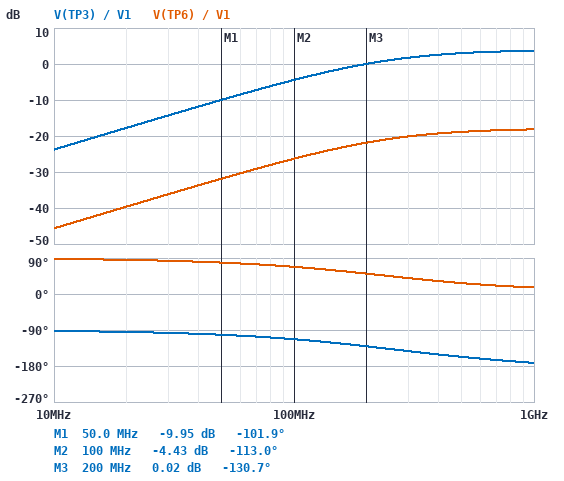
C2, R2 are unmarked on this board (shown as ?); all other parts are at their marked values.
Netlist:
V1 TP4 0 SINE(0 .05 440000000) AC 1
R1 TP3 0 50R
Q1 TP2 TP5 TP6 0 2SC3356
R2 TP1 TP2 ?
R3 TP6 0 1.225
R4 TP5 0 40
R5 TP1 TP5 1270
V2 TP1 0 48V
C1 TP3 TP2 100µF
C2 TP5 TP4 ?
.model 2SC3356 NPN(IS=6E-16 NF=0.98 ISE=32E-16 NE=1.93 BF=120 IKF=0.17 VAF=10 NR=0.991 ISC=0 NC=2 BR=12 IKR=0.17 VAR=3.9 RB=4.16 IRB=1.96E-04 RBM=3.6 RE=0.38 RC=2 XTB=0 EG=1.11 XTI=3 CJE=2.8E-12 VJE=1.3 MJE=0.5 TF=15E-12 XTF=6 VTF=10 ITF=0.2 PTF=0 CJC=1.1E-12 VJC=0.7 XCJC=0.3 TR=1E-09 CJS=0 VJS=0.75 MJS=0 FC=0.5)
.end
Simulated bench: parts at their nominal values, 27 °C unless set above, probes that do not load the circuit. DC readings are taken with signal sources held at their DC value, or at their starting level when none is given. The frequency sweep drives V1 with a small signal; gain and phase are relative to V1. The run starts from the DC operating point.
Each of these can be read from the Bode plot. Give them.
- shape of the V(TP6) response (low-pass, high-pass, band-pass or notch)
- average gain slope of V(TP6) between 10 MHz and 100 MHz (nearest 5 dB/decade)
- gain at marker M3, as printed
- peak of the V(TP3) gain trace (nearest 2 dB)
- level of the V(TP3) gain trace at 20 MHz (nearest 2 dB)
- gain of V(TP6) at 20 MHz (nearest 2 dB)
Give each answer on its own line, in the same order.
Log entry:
high-pass
20 dB/decade
0.02 dB
4 dB
-18 dB
-40 dB
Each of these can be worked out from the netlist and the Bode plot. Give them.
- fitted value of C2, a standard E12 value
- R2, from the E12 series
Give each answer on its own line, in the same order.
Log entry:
3.3 pF
22 Ω
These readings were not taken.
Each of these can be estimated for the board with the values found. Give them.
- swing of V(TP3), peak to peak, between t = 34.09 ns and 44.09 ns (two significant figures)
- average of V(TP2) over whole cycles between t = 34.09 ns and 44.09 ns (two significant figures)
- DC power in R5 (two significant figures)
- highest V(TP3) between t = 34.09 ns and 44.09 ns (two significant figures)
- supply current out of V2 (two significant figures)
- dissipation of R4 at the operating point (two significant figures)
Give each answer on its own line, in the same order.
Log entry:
140 mV
40 V
1.7 W
69 mV
400 mA
51 mW
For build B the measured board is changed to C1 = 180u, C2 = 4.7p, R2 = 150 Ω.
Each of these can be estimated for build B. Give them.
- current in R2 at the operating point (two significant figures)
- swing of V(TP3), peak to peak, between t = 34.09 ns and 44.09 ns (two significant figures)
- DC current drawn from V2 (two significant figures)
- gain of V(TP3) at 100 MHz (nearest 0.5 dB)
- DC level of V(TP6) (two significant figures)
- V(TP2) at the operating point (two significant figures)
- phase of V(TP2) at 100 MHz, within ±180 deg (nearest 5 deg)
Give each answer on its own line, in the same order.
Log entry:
270 mA
100 mV
310 mA
-2.0 dB
340 mV
7.4 V
-140 deg
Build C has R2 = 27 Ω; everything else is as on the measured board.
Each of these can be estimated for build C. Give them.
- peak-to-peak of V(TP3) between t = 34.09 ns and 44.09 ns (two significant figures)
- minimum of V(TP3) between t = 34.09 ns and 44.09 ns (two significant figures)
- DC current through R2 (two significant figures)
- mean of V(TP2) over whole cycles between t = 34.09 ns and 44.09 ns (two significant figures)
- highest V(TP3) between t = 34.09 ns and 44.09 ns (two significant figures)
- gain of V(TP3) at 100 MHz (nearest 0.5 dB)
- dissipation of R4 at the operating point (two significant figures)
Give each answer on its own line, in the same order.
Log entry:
150 mV
-76 mV
360 mA
38 V
76 mV
-3.5 dB
51 mW
